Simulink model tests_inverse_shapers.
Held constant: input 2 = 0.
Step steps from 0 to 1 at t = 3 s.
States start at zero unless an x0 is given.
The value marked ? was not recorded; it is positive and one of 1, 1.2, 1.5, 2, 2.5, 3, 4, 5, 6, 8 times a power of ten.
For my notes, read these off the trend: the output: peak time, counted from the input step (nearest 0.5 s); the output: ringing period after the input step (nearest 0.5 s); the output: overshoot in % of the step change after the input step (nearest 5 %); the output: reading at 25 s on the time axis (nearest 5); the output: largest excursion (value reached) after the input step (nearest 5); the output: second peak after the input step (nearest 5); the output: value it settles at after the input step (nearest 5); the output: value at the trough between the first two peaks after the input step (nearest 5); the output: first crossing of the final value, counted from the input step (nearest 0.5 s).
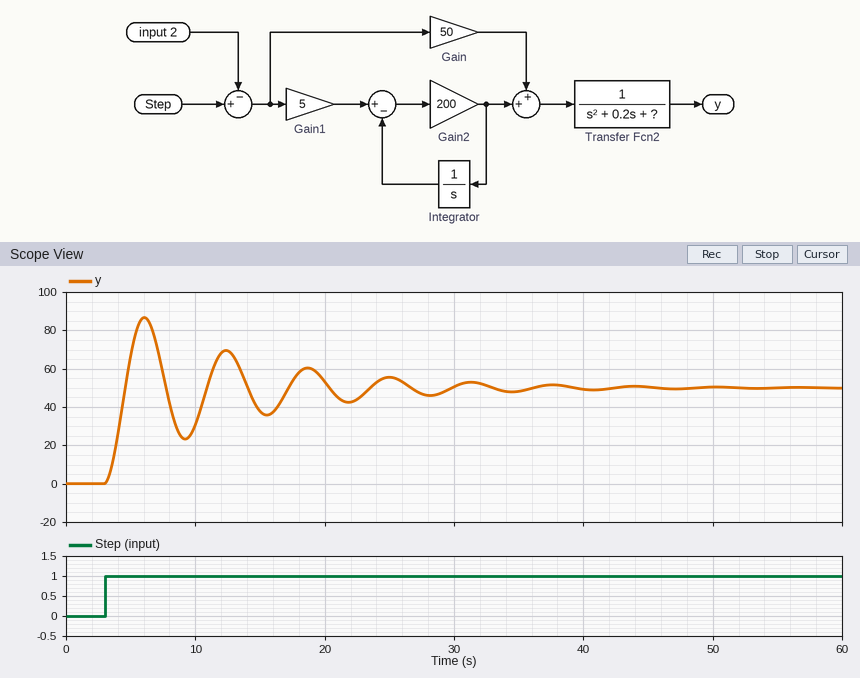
3.0 s
6.5 s
75 %
55
85
70
50
25
1.5 s
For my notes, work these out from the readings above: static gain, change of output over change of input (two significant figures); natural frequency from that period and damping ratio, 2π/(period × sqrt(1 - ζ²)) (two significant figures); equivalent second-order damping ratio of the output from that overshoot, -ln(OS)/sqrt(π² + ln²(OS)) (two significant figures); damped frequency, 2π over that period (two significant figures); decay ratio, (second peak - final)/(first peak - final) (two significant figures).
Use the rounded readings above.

50
0.97 rad/s
0.091
0.97 rad/s
0.57
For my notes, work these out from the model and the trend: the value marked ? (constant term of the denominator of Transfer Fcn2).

1
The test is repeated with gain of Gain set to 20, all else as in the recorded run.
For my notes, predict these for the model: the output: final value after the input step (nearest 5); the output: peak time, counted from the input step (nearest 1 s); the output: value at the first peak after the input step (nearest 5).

20
3 s
35
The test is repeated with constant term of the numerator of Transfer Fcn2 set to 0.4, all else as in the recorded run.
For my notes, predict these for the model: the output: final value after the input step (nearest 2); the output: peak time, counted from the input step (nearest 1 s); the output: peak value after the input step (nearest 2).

20
3 s
34
